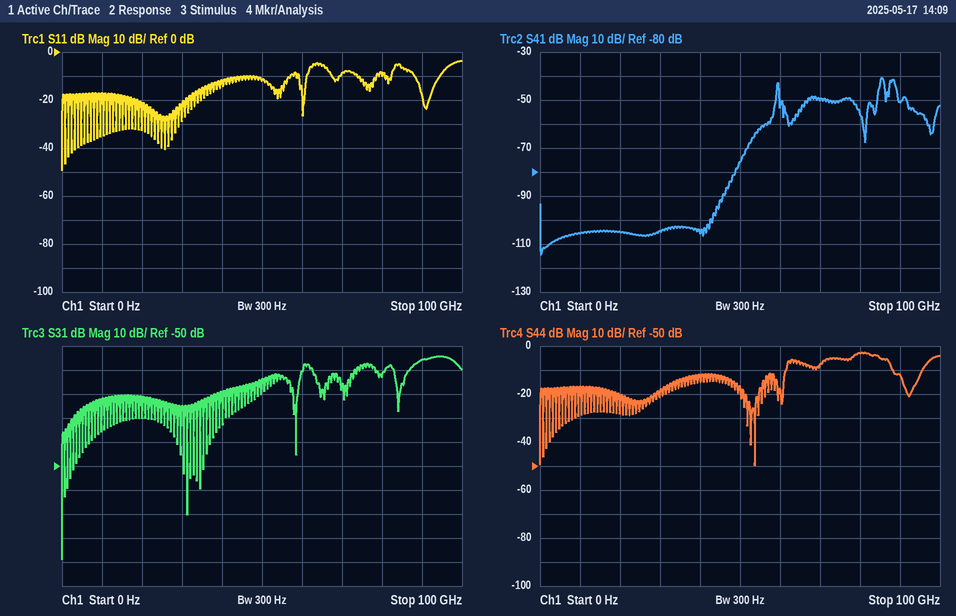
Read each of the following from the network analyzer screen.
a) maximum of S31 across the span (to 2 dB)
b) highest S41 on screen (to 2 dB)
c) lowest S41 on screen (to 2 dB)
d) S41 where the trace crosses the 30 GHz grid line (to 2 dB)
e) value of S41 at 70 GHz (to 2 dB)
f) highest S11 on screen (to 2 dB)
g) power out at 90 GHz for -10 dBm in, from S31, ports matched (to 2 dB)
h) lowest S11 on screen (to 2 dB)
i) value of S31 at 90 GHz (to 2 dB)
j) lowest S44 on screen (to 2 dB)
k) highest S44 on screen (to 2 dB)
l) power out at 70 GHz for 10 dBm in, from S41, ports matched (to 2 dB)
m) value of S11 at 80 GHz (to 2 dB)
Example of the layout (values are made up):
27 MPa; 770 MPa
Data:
-4 dB; -40 dB; -114 dB; -104 dB; -50 dB; -4 dB; -16 dBm; -50 dB; -6 dB; -50 dB; -2 dB; -40 dBm; -10 dB
